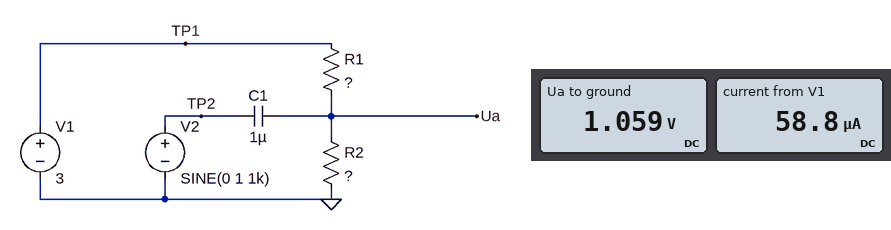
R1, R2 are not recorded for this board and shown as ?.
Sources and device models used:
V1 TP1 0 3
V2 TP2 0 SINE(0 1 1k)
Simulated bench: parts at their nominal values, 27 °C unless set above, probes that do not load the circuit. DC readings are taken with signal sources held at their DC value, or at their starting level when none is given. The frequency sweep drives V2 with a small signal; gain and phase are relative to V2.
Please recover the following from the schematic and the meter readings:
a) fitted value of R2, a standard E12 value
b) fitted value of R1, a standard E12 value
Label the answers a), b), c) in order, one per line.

a) 18 kΩ
b) 33 kΩ
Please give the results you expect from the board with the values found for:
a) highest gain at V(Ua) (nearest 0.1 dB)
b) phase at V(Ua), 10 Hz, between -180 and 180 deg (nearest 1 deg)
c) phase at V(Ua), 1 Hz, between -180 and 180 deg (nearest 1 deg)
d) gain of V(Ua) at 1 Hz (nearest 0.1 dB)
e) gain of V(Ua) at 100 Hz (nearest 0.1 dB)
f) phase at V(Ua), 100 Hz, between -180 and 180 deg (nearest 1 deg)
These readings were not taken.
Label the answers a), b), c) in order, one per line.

a) 0 dB
b) 54 deg
c) 86 deg
d) -22.7 dB
e) -0.1 dB
f) 8 deg
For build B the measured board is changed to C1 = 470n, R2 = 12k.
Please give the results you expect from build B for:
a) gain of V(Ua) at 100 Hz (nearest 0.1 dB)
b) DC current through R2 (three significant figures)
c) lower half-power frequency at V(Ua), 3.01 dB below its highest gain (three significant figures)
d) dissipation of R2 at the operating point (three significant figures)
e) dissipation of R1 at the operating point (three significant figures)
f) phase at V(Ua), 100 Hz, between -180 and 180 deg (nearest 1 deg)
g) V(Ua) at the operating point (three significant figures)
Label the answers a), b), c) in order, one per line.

a) -0.6 dB
b) 66.7 µA
c) 38.5 Hz
d) 53.3 µW
e) 147 µW
f) 21 deg
g) 800 mV
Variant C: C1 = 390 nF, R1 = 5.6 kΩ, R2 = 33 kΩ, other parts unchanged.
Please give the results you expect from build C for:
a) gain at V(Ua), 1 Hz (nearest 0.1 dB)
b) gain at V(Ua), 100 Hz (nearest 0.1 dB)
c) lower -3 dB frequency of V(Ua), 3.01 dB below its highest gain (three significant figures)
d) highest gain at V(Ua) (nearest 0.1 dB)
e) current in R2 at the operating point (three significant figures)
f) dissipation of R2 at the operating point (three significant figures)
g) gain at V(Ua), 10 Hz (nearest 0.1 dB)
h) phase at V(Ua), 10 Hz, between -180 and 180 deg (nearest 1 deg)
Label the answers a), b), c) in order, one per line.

a) -38.6 dB
b) -2.4 dB
c) 85.2 Hz
d) 0 dB
e) 77.7 µA
f) 199 µW
g) -18.7 dB
h) 83 deg
